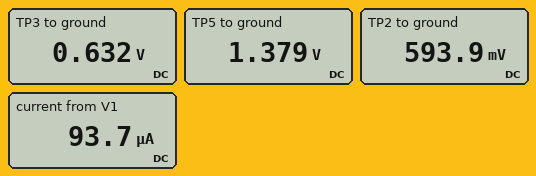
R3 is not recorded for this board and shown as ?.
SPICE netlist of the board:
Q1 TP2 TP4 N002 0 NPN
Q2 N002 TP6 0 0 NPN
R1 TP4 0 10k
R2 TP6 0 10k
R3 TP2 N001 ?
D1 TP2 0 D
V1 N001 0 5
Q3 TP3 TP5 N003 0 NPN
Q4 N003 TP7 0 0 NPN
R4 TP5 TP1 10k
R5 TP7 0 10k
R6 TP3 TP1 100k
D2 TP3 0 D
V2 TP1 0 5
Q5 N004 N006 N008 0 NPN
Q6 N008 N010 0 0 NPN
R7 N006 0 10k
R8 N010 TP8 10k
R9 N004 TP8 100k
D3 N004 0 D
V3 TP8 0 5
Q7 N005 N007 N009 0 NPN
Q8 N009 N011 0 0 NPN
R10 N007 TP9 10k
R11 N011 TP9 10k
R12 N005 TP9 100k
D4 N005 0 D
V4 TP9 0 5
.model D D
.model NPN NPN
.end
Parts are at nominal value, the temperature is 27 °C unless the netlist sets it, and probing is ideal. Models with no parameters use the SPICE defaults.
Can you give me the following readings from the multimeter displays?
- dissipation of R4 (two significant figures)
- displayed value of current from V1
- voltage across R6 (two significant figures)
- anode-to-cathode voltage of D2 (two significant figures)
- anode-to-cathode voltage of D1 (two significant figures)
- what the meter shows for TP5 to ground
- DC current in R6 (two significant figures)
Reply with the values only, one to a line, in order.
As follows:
1.3 mW
93.7 µA
4.4 V
630 mV
590 mV
1.379 V
44 µA
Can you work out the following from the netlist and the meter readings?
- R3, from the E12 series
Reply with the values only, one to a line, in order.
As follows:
47 kΩ
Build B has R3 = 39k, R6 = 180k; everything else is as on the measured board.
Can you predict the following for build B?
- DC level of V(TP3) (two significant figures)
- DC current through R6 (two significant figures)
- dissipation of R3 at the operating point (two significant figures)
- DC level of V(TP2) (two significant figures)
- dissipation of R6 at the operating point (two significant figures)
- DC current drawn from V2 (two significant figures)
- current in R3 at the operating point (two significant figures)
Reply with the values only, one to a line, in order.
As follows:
630 mV
24 µA
500 µW
600 mV
110 µW
390 µA
110 µA
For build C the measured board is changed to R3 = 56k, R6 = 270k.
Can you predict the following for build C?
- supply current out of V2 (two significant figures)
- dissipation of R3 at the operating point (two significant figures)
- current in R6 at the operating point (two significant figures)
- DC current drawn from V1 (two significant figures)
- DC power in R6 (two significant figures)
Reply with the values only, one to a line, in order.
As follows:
380 µA
350 µW
16 µA
79 µA
71 µW
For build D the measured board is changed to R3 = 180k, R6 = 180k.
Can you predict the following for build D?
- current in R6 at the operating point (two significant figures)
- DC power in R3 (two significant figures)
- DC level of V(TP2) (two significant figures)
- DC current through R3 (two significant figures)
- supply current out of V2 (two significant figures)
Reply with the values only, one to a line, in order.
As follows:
24 µA
110 µW
560 mV
25 µA
390 µA
